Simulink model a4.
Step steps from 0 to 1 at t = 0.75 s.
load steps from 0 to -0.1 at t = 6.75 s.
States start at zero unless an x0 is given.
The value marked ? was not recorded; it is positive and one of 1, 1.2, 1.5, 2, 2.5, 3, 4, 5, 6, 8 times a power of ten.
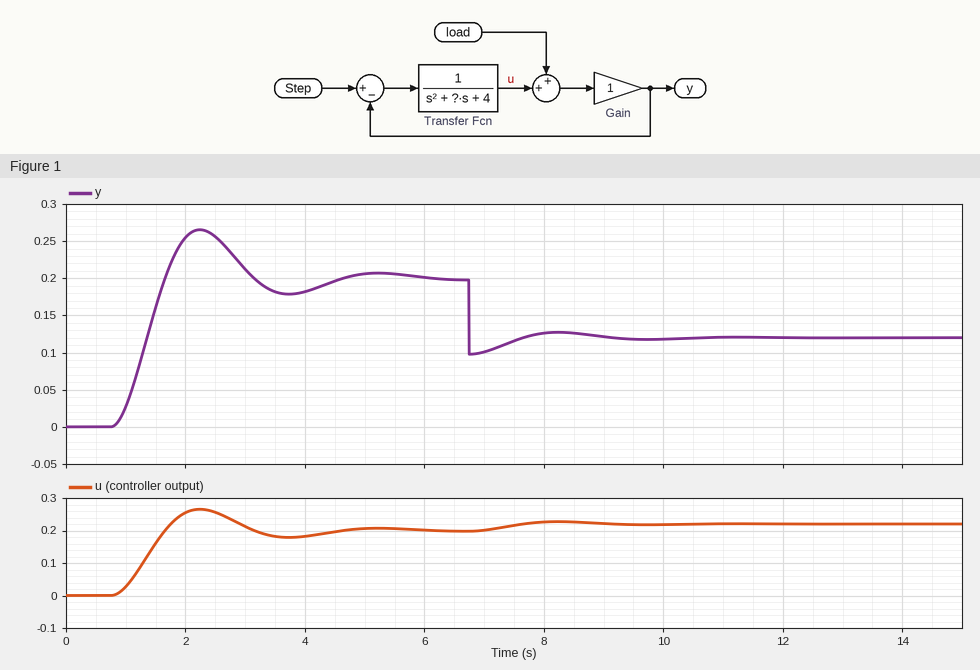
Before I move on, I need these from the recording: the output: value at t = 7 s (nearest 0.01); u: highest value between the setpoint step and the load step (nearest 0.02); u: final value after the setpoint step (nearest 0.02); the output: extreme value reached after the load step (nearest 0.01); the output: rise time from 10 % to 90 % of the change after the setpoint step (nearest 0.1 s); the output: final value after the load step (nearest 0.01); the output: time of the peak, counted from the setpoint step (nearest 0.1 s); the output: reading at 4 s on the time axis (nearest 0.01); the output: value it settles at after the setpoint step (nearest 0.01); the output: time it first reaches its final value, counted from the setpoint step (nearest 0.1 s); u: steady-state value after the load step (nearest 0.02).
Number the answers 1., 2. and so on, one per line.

1. 0.10
2. 0.26
3. 0.20
4. 0.10
5. 0.6 s
6. 0.12
7. 1.5 s
8. 0.18
9. 0.20
10. 0.9 s
11. 0.22
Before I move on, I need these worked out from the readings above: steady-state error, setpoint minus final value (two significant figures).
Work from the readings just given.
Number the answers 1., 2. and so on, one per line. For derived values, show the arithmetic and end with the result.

1. 1 - 0.2 = 0.80
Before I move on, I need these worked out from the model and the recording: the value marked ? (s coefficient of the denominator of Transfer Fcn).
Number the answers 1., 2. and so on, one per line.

1. 1.5
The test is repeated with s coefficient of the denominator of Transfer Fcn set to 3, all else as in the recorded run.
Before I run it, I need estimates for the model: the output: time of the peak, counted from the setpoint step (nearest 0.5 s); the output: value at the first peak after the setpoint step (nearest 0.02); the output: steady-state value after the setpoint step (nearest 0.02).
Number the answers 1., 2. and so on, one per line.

1. 2.0 s
2. 0.22
3. 0.20
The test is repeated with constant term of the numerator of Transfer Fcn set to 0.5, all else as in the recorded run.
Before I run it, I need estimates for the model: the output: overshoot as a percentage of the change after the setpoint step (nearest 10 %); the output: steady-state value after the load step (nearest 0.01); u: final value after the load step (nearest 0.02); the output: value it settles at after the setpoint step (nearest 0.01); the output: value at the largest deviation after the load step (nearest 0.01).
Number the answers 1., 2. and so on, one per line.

1. 30 %
2. 0.02
3. 0.12
4. 0.11
5. 0.01
